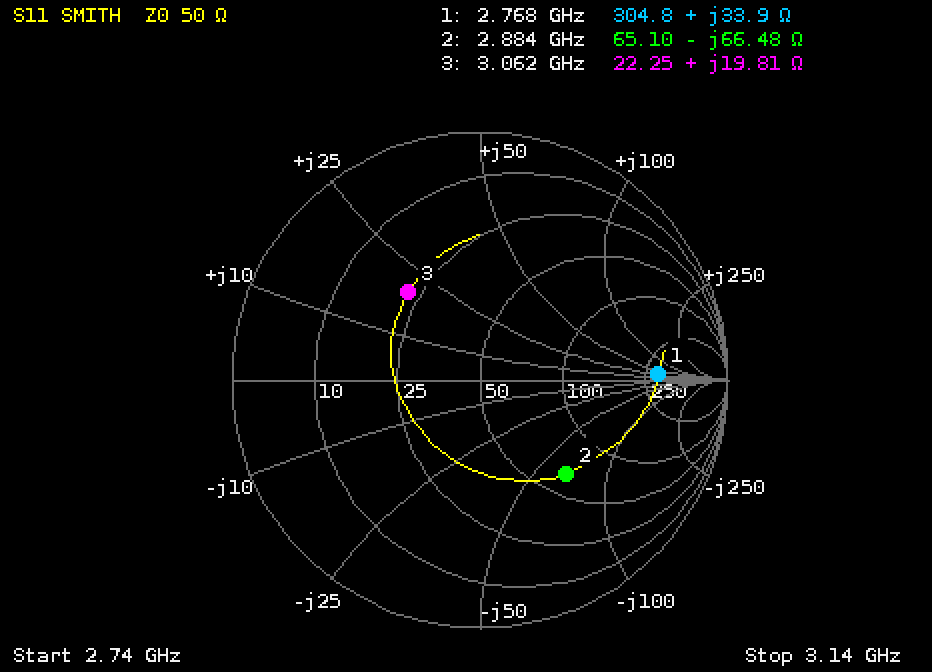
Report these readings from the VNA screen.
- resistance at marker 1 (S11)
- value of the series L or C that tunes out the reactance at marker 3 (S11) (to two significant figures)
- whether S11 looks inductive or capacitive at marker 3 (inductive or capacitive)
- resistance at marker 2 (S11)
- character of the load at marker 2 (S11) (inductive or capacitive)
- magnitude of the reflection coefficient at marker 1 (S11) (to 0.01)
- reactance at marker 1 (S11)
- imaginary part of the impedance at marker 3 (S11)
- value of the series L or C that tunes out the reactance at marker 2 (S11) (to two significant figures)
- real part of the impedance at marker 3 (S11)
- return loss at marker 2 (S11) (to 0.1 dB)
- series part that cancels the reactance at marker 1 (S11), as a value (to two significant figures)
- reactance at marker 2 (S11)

304.8 Ω
2.6 pF
inductive
65.10 Ω
capacitive
0.72
+33.9 Ω
+19.81 Ω
3.7 nH
22.25 Ω
5.8 dB
1.7 pF
-66.48 Ω
